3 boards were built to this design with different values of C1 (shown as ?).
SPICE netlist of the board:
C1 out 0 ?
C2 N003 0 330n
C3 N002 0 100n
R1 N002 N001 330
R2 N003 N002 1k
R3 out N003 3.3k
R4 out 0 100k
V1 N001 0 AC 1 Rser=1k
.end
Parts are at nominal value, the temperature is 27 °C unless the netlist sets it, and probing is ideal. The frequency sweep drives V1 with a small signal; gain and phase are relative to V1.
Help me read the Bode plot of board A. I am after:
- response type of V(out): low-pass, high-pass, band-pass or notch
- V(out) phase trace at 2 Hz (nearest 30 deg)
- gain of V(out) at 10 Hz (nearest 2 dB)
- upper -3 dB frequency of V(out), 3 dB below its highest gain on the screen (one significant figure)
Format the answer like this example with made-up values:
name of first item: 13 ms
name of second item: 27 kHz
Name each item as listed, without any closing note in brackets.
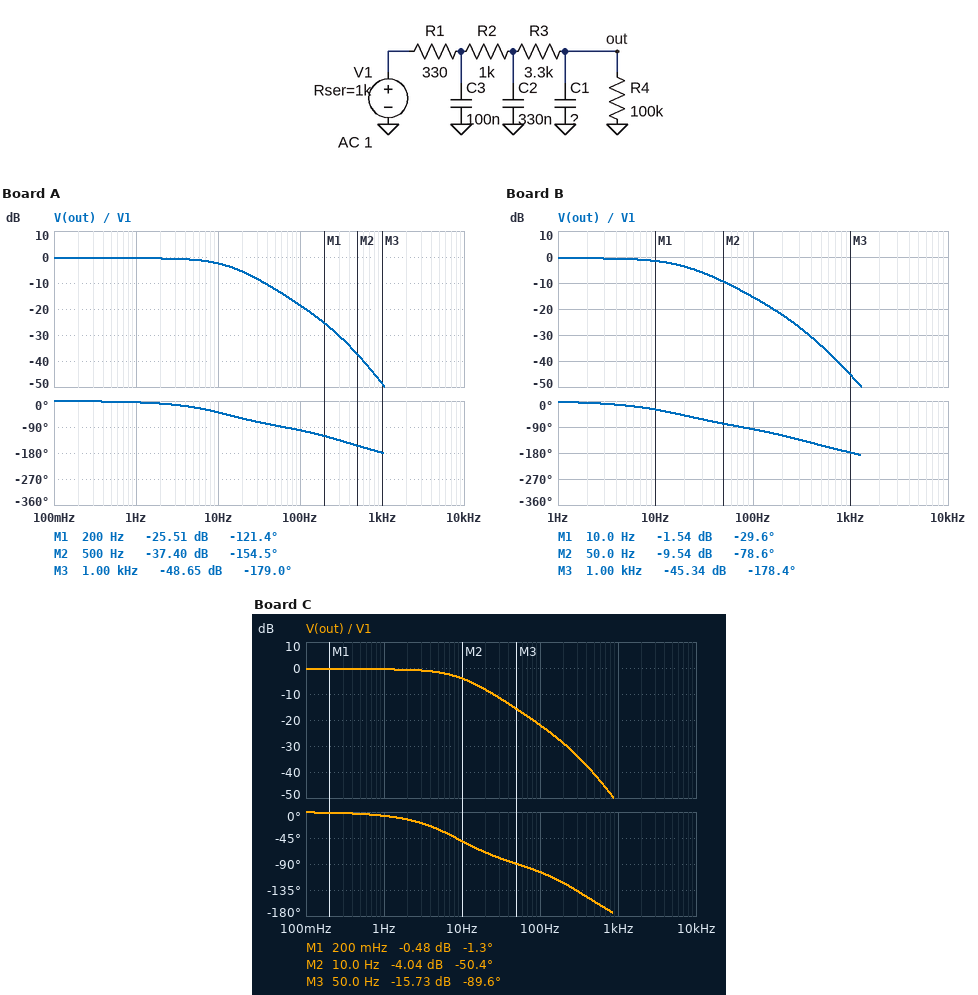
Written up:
response type of V(out): low-pass, high-pass, band-pass or notch: low-pass
V(out) phase trace at 2 Hz: 0 deg
gain of V(out) at 10 Hz: -2 dB
upper -3 dB frequency of V(out), 3 dB below its highest gain on the screen: 10 Hz
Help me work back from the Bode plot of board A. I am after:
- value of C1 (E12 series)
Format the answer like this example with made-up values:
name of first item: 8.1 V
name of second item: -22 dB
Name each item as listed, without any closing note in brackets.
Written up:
value of C1: 2.2 µF
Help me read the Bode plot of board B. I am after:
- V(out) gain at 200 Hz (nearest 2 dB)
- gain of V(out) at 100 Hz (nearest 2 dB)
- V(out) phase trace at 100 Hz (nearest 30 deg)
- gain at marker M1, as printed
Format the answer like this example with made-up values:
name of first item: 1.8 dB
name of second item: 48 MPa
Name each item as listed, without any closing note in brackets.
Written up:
V(out) gain at 200 Hz: -22 dB
gain of V(out) at 100 Hz: -16 dB
V(out) phase trace at 100 Hz: -90 deg
gain at marker M1, as printed: -1.54 dB
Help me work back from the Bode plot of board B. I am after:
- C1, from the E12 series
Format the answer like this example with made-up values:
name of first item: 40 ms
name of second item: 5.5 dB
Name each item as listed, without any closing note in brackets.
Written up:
C1, from the E12 series: 1.5 µF
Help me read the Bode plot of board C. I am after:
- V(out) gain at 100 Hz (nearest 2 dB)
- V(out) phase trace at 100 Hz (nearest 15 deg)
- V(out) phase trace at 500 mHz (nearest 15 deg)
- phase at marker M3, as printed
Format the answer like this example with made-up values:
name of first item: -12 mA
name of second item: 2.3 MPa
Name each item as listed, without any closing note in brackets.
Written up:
V(out) gain at 100 Hz: -22 dB
V(out) phase trace at 100 Hz: -105 deg
V(out) phase trace at 500 mHz: 0 deg
phase at marker M3, as printed: -89.6 deg
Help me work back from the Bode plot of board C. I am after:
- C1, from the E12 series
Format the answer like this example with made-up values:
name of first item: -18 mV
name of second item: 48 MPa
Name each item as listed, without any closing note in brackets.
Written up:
C1, from the E12 series: 3.3 µF
